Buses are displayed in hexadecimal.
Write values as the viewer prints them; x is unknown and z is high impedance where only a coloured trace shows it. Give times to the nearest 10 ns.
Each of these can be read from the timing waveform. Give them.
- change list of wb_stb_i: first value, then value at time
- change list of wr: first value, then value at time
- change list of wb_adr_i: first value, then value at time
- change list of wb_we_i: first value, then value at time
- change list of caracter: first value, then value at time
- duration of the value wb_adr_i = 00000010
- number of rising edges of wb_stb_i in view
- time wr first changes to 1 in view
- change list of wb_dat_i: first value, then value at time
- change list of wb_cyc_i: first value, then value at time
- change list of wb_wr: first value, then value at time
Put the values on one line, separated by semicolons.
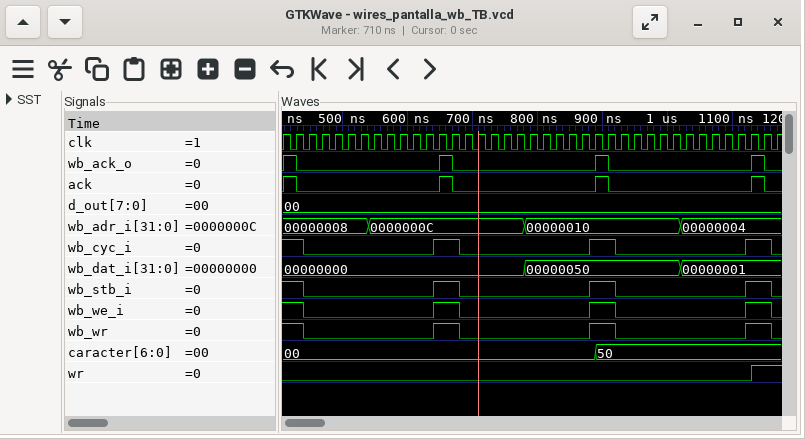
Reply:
1, 0 at 440 ns, 1 at 640 ns, 0 at 680 ns, 1 at 880 ns, 0 at 920 ns, 1 at 1120 ns, 0 at 1160 ns; 0, 1 at 1130 ns; 00000008, 0000000C at 540 ns, 00000010 at 780 ns, 00000004 at 1020 ns; 1, 0 at 440 ns, 1 at 640 ns, 0 at 680 ns, 1 at 880 ns, 0 at 920 ns, 1 at 1120 ns, 0 at 1160 ns; 00, 50 at 890 ns; 240 ns; 3; 1130 ns; 00000000, 00000050 at 780 ns, 00000001 at 1020 ns; 1, 0 at 440 ns, 1 at 640 ns, 0 at 680 ns, 1 at 880 ns, 0 at 920 ns, 1 at 1120 ns, 0 at 1160 ns; 1, 0 at 440 ns, 1 at 640 ns, 0 at 680 ns, 1 at 880 ns, 0 at 920 ns, 1 at 1120 ns, 0 at 1160 ns
